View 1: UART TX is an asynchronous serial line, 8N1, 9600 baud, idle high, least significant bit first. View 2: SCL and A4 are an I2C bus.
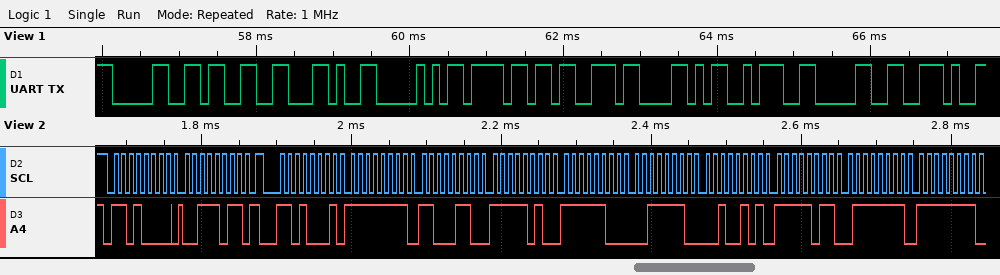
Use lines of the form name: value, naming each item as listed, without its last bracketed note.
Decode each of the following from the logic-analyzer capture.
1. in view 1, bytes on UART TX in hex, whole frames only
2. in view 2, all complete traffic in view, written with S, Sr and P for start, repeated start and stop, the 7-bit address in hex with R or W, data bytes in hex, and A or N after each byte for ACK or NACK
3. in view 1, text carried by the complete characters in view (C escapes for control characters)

in view 1, bytes on UART TX in hex, whole frames only: 0x30 0x33 0x2C 0x50 0x6F 0x73 0x58 0x3A 0x30 0x2E
in view 2, all complete traffic in view, written with S, Sr and P for start, repeated start and stop, the 7-bit address in hex with R or W, data bytes in hex, and A or N after each byte for ACK or NACK: S 68W A 3B A Sr 68R A FF A C6 A FA A FC A 3E A 25 A FB A 7F A FF A
in view 1, text carried by the complete characters in view: "03,PosX:0."
